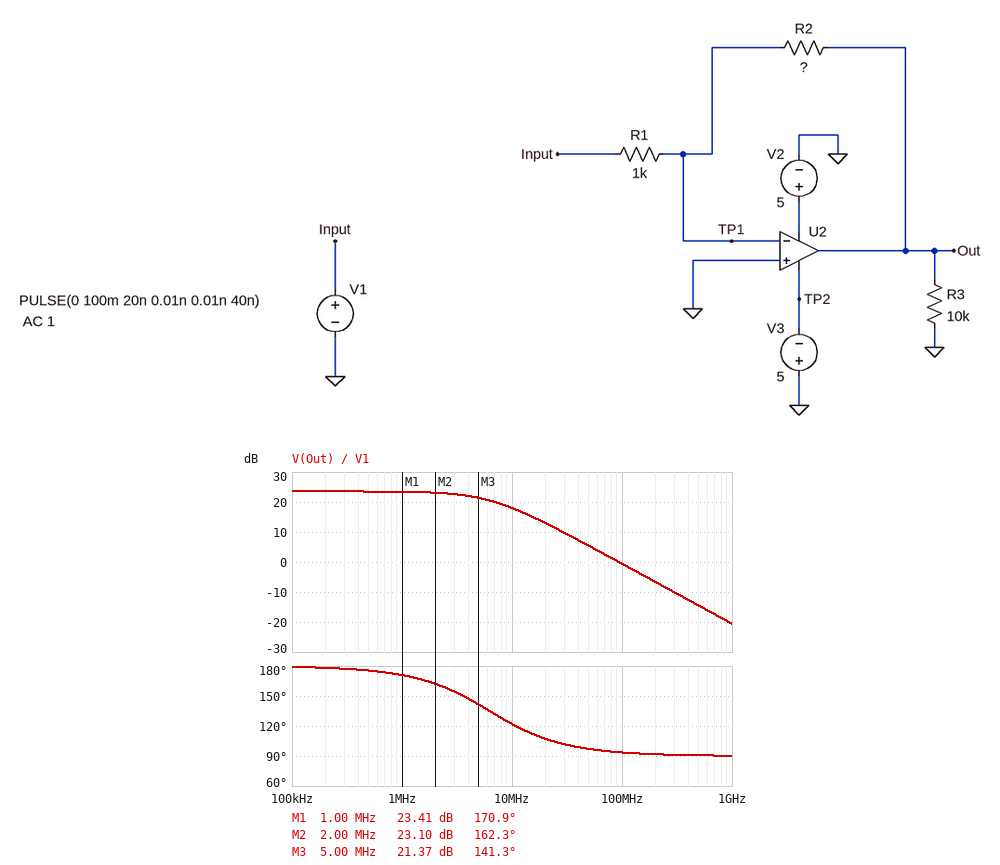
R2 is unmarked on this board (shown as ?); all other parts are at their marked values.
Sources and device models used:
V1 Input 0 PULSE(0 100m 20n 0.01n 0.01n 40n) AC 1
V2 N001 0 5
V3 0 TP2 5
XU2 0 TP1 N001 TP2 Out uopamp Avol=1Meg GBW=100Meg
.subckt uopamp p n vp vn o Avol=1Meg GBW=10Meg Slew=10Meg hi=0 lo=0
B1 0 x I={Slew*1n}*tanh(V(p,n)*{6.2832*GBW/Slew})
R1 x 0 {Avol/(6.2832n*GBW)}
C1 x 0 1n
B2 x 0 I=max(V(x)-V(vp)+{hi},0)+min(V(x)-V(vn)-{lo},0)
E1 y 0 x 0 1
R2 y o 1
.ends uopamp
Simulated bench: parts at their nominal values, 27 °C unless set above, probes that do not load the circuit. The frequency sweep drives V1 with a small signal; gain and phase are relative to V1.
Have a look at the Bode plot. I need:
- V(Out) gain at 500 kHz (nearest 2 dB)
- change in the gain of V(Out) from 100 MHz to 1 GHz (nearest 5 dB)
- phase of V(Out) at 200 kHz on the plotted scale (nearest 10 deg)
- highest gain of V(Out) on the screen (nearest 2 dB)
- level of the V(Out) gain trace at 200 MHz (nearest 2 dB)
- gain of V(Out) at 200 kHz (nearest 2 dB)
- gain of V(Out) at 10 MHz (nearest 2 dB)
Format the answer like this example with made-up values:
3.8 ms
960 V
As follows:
24 dB
-20 dB
180 deg
24 dB
-6 dB
24 dB
18 dB
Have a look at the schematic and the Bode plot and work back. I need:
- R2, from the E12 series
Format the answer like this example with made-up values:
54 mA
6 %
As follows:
15 kΩ
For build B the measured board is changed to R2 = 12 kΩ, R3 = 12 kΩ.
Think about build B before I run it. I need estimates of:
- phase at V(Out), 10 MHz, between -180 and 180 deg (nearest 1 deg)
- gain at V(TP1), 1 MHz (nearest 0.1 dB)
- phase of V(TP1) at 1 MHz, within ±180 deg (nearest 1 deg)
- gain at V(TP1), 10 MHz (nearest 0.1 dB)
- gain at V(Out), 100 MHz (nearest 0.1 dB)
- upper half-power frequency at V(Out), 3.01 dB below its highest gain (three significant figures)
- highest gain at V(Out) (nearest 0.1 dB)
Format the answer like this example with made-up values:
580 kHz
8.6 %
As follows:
128 deg
-18.5 dB
83 deg
-2.7 dB
-0.7 dB
7.69 MHz
21.6 dB
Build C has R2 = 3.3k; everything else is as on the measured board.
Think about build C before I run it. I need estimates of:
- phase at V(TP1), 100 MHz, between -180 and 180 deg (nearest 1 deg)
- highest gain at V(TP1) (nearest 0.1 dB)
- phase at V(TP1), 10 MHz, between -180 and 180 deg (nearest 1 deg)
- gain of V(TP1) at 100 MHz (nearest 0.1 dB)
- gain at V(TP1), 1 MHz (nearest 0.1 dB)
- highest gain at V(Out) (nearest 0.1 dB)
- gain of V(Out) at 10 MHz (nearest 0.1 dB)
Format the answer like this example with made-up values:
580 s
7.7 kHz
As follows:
13 deg
-2.3 dB
67 deg
-2.5 dB
-29.6 dB
10.4 dB
9.6 dB
